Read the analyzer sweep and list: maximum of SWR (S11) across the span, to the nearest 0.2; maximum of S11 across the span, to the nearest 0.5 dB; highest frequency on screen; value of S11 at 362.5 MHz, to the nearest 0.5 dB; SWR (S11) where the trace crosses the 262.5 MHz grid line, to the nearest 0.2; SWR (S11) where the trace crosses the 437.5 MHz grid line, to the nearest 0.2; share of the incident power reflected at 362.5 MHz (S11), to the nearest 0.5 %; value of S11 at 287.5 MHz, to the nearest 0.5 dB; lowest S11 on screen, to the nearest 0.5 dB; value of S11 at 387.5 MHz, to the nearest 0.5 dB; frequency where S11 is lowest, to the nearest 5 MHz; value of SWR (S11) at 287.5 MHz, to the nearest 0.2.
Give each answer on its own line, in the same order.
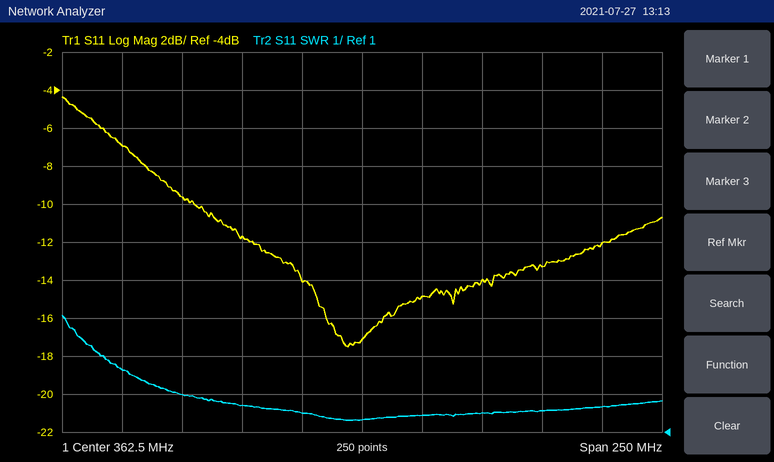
4.0
-4.5 dB
487.5 MHz
-17.0 dB
2.6
1.6
2.0 %
-9.5 dB
-17.5 dB
-15.0 dB
355 MHz
2.0
